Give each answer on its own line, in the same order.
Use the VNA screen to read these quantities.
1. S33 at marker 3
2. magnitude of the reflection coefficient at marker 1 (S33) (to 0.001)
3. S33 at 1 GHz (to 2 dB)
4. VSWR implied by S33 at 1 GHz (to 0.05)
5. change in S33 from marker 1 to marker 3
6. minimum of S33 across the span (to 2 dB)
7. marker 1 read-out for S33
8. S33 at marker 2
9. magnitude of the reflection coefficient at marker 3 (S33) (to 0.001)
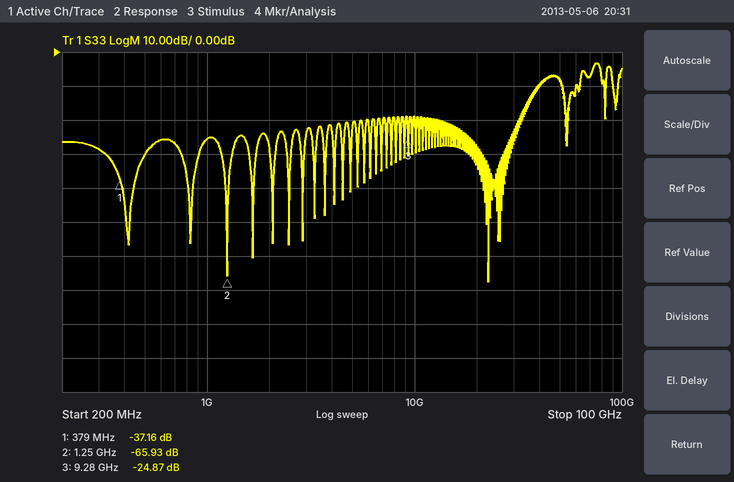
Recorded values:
-24.87 dB
0.014
-26 dB
1.10
12.29 dB
-68 dB
-37.16 dB
-65.93 dB
0.057
